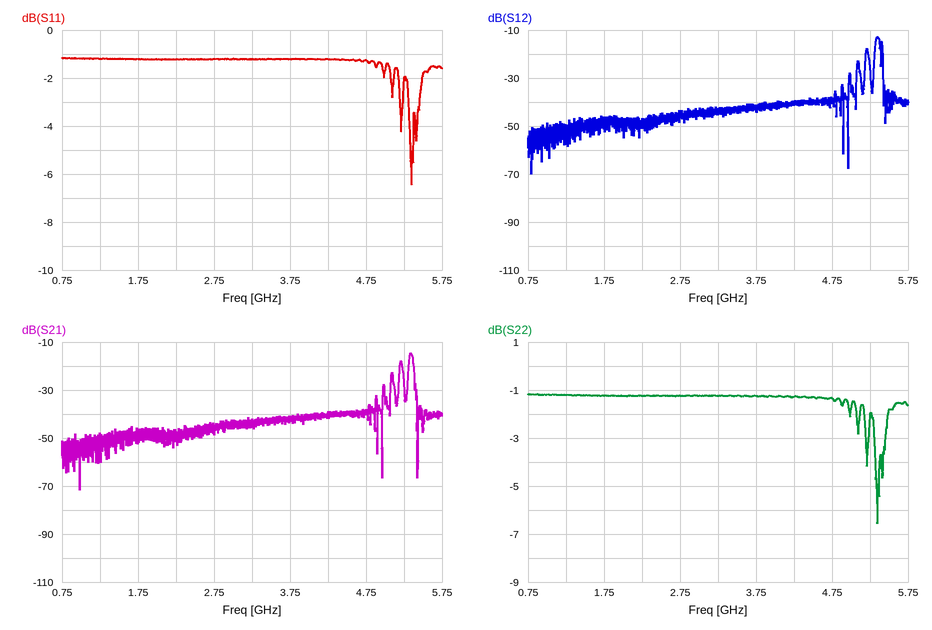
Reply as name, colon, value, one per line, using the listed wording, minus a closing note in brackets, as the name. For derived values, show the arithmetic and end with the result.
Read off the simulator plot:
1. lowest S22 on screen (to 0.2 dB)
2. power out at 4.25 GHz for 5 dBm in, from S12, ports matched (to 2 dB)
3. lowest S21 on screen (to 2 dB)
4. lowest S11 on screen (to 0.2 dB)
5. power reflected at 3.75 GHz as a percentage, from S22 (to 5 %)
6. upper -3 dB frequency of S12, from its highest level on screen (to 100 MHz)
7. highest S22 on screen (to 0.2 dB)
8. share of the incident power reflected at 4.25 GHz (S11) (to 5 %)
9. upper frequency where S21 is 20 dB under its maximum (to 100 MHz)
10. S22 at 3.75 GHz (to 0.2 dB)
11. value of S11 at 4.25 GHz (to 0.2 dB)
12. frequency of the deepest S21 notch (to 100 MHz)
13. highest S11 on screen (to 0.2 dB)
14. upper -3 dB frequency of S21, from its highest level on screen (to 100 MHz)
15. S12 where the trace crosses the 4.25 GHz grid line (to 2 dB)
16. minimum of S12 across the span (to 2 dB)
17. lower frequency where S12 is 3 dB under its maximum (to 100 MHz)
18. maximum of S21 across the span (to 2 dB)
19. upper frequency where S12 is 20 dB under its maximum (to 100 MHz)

lowest S22 on screen: -6.6 dB
power out at 4.25 GHz for 5 dBm in, from S12, ports matched: 5 dBm + (-40 dB) = -36 dBm
lowest S21 on screen: -72 dB
lowest S11 on screen: -6.4 dB
power reflected at 3.75 GHz as a percentage, from S22: 10^(-1.2/10) ≈ 75.9 %, so 75 % to the nearest 5 %
upper -3 dB frequency of S12, from its highest level on screen: 5.4 GHz
highest S22 on screen: -1.2 dB
share of the incident power reflected at 4.25 GHz (S11): 10^(-1.2/10) ≈ 75.9 %, so 75 % to the nearest 5 %
upper frequency where S21 is 20 dB under its maximum: 5.4 GHz
S22 at 3.75 GHz: -1.2 dB
value of S11 at 4.25 GHz: -1.2 dB
frequency of the deepest S21 notch: 1.0 GHz
highest S11 on screen: -1.2 dB
upper -3 dB frequency of S21, from its highest level on screen: 5.4 GHz
S12 where the trace crosses the 4.25 GHz grid line: -40 dB
minimum of S12 across the span: -70 dB
lower frequency where S12 is 3 dB under its maximum: 5.3 GHz
maximum of S21 across the span: -14 dB
upper frequency where S12 is 20 dB under its maximum: 5.4 GHz
